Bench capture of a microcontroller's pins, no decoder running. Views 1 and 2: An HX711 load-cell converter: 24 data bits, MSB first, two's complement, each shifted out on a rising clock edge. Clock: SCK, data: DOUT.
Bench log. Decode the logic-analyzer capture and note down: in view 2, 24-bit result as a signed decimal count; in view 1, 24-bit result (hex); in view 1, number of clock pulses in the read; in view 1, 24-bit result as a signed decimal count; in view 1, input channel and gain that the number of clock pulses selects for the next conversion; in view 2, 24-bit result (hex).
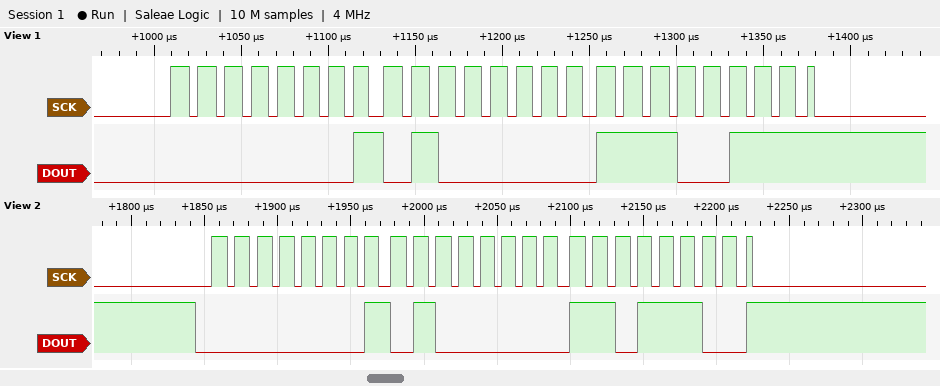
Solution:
82140
0x0140E7
25
82151
channel A, gain 128
0x0140DC
